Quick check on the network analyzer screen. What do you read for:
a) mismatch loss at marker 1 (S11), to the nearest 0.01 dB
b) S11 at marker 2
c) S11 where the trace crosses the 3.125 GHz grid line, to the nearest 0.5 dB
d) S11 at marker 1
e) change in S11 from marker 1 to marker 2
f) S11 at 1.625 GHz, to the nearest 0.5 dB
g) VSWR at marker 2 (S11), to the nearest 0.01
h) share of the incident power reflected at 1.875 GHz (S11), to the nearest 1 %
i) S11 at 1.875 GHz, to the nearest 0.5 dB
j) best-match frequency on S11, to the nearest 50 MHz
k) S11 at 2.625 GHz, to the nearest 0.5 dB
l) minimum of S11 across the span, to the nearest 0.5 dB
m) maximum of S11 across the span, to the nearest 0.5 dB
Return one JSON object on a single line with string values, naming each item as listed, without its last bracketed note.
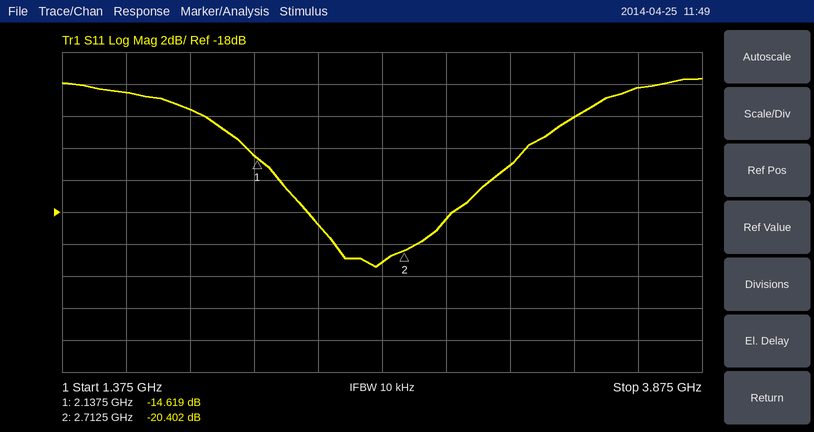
{"mismatch loss at marker 1 (S11), to the nearest 0.01 dB": "0.15 dB", "S11 at marker 2": "-20.402 dB", "S11 where the trace crosses the 3.125 GHz grid line, to the nearest 0.5 dB": "-15.0 dB", "S11 at marker 1": "-14.619 dB", "change in S11 from marker 1 to marker 2": "-5.783 dB", "S11 at 1.625 GHz, to the nearest 0.5 dB": "-10.5 dB", "VSWR at marker 2 (S11), to the nearest 0.01": "1.21", "share of the incident power reflected at 1.875 GHz (S11), to the nearest 1 %": "7 %", "S11 at 1.875 GHz, to the nearest 0.5 dB": "-11.5 dB", "best-match frequency on S11, to the nearest 50 MHz": "2.60 GHz", "S11 at 2.625 GHz, to the nearest 0.5 dB": "-21.0 dB", "minimum of S11 across the span, to the nearest 0.5 dB": "-21.5 dB", "maximum of S11 across the span, to the nearest 0.5 dB": "-9.5 dB"}
